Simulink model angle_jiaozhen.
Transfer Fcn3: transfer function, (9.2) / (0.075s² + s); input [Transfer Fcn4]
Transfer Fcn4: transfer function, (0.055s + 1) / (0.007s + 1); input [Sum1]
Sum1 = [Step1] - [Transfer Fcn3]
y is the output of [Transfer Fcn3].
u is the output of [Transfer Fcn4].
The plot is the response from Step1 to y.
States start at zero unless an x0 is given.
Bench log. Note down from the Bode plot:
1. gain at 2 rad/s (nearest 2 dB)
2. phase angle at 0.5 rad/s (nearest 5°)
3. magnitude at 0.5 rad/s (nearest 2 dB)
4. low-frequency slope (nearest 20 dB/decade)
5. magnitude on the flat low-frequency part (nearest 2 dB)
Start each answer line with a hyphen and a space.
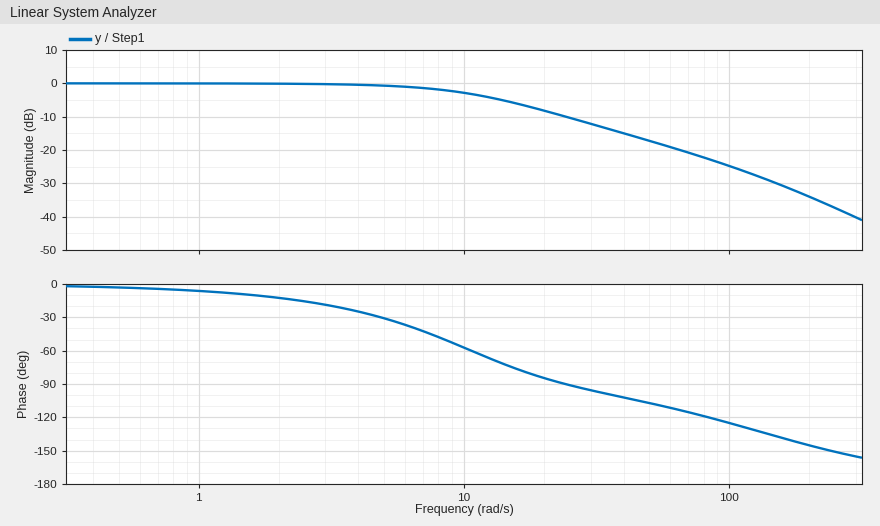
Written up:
- 0 dB
- -5°
- 0 dB
- 0 dB/decade
- 0 dB
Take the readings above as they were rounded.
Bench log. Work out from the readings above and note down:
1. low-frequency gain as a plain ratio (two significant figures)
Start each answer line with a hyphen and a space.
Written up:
- 1.0
